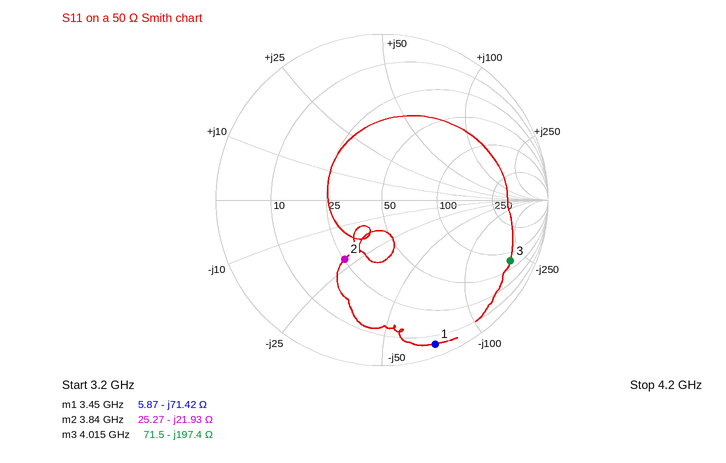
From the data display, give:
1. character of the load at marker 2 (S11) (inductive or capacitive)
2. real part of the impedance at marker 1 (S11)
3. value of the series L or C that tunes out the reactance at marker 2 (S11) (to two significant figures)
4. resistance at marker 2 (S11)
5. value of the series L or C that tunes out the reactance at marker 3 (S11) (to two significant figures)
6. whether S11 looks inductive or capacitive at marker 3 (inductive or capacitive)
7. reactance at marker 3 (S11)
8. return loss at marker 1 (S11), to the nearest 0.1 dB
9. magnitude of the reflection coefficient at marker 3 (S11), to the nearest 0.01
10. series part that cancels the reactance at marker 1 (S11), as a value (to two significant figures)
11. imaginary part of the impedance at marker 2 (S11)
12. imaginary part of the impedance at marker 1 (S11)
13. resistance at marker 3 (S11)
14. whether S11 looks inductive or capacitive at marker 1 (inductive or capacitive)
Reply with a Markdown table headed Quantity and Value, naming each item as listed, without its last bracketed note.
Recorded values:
| Quantity | Value |
|---|---|
| character of the load at marker 2 (S11) | capacitive |
| real part of the impedance at marker 1 | 5.87 Ω |
| value of the series L or C that tunes out the reactance at marker 2 (S11) | 910 pH |
| resistance at marker 2 | 25.27 Ω |
| value of the series L or C that tunes out the reactance at marker 3 (S11) | 7.8 nH |
| whether S11 looks inductive or capacitive at marker 3 | capacitive |
| reactance at marker 3 | -197.4 Ω |
| return loss at marker 1 (S11), to the nearest 0.1 dB | 0.7 dB |
| magnitude of the reflection coefficient at marker 3 (S11), to the nearest 0.01 | 0.86 |
| series part that cancels the reactance at marker 1 (S11), as a value | 3.3 nH |
| imaginary part of the impedance at marker 2 | -21.93 Ω |
| imaginary part of the impedance at marker 1 | -71.42 Ω |
| resistance at marker 3 | 71.5 Ω |
| whether S11 looks inductive or capacitive at marker 1 | capacitive |
